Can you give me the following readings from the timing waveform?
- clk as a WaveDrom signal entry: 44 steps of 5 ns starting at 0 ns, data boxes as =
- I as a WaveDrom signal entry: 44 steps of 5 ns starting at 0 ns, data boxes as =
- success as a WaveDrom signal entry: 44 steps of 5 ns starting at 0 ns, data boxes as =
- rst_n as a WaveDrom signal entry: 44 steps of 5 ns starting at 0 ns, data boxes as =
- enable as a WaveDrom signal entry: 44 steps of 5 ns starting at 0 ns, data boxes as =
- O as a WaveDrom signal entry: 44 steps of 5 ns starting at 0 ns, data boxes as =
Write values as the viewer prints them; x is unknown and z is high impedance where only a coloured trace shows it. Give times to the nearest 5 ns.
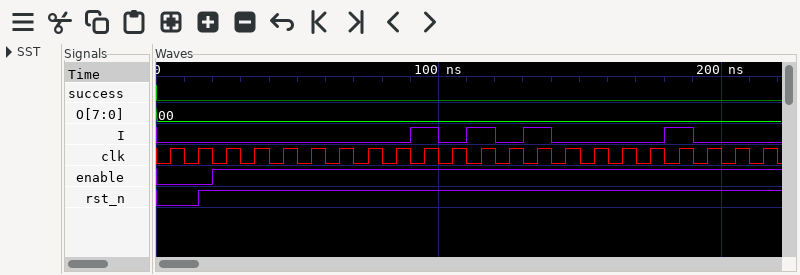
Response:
{name: 'clk', wave: '01010101010101010101010101010101010101010101'}
{name: 'I', wave: '0.................1.0.1.0.1.0.......1.0.....'}
{name: 'success', wave: '0...........................................'}
{name: 'rst_n', wave: '0..1........................................'}
{name: 'enable', wave: '0...1.......................................'}
{name: 'O', wave: '=...........................................', data: '00'}
